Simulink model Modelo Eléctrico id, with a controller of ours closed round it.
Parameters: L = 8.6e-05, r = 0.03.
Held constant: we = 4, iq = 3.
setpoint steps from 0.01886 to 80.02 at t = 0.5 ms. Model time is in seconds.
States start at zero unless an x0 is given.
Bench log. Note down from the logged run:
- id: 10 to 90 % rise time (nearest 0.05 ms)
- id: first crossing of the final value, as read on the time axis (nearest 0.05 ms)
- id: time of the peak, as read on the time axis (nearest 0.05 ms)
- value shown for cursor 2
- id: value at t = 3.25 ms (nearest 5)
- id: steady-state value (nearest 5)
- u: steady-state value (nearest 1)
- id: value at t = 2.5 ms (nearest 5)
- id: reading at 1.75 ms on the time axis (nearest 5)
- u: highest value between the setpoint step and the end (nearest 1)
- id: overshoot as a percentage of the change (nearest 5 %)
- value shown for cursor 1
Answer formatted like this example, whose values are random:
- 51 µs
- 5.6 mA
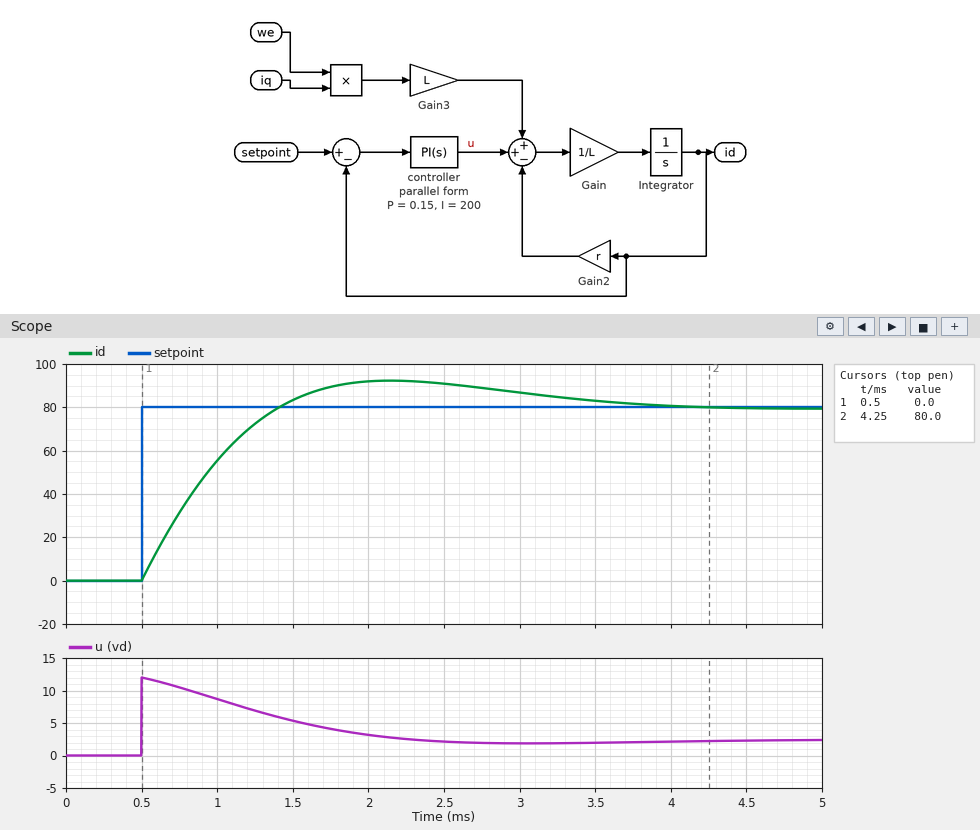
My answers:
- 0.70 ms
- 1.40 ms
- 2.15 ms
- 80.0
- 85
- 80
- 2
- 90
- 90
- 12
- 15 %
- 0.0
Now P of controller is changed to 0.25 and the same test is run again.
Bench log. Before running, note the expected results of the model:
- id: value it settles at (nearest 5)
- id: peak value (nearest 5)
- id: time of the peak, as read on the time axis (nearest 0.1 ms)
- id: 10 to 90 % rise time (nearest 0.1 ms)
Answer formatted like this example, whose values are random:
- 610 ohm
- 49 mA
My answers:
- 80
- 85
- 2.0 ms
- 0.6 ms
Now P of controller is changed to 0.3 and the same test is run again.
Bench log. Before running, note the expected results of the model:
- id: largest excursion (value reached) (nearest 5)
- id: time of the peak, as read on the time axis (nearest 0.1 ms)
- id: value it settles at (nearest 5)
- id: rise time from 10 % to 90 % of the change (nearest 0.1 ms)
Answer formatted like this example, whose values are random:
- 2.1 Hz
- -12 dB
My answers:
- 85
- 1.9 ms
- 80
- 0.5 ms
